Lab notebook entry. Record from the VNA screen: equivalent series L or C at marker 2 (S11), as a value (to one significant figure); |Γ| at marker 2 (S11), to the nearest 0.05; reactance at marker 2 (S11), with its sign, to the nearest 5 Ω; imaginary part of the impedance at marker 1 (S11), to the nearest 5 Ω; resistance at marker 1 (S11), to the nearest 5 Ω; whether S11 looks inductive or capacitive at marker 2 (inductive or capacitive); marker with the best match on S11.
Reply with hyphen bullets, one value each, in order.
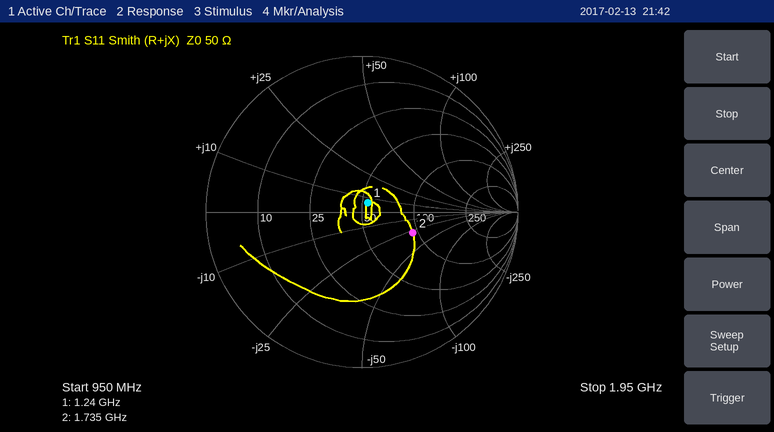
- 3 pF
- 0.35
- -30 Ω
- +5 Ω
- 55 Ω
- capacitive
- marker 1
